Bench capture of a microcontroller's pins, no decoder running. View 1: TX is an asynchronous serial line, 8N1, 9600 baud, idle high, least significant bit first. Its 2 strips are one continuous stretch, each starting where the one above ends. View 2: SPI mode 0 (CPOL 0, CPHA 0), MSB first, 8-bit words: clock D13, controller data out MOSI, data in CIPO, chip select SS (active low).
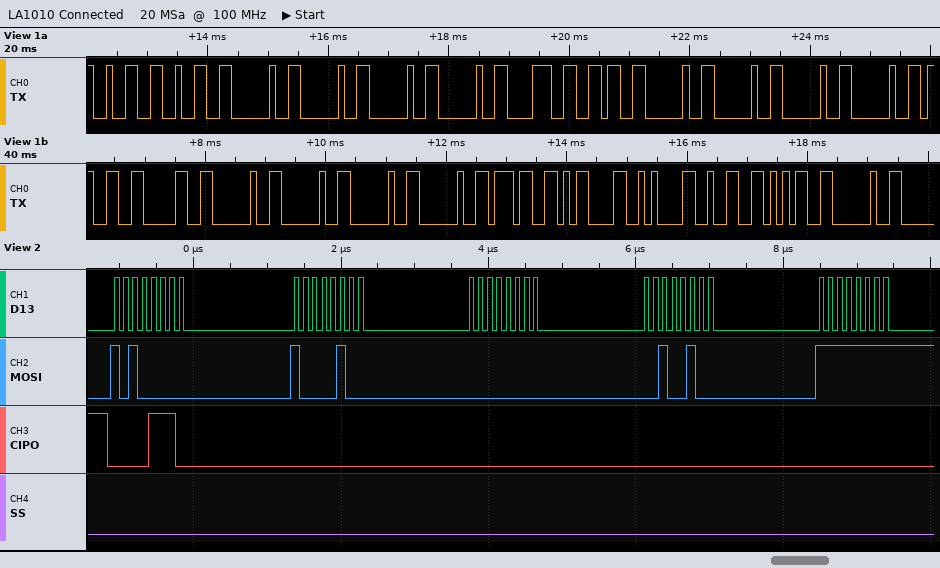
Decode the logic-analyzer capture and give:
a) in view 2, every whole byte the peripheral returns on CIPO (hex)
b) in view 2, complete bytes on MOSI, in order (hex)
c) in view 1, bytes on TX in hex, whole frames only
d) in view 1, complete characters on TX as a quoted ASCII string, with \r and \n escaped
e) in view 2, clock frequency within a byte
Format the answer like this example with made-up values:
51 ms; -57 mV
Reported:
0E 00 00 00 00; A0 84 00 24 FF; 0x32 0x32 0x20 0x20 0x20 0x20 0x38 0x36 0x20 0x20 0x20 0x20 0x33 0x30 0x20 0x20 0x20 0x20 0x37 0x0D 0x0A 0x32 0x35 0x20; "22    86    30    7\r\n25 "; 8 MHz
